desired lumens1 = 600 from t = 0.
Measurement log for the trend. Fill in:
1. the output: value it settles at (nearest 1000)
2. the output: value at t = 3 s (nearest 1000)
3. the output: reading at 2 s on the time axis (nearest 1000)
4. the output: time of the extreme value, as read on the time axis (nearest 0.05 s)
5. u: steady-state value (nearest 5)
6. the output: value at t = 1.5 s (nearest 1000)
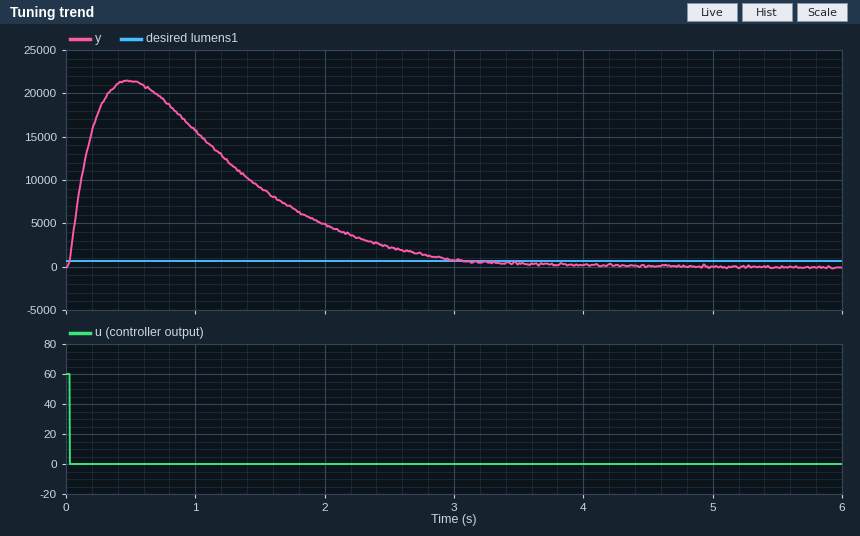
0
1000
5000
0.50 s
0
9000
